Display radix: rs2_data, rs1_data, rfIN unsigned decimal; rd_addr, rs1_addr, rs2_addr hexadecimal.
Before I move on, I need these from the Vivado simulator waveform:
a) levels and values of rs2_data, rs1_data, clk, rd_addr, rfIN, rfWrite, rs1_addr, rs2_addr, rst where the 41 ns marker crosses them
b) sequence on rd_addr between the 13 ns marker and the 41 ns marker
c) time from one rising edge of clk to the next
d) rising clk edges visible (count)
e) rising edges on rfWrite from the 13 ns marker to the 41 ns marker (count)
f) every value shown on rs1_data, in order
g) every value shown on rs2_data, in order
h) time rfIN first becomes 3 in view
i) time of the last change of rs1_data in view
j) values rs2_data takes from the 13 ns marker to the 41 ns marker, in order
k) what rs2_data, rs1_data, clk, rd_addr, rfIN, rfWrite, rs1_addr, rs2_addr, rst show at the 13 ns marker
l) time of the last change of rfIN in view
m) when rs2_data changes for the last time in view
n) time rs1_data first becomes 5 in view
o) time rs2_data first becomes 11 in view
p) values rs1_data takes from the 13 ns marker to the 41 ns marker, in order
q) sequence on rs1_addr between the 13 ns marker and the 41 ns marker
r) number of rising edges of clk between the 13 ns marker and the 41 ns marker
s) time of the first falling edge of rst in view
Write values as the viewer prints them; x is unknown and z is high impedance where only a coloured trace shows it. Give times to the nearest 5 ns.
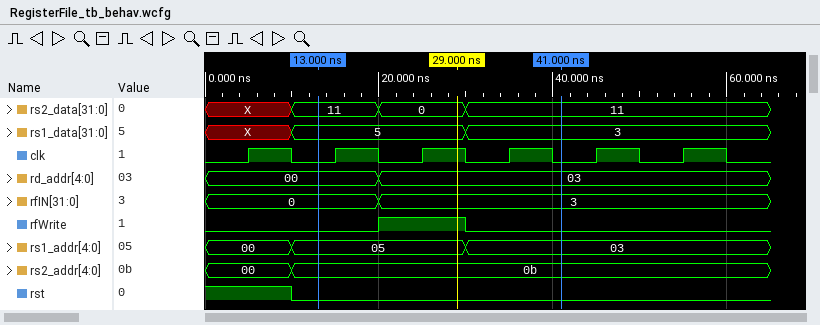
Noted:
rs2_data=11, rs1_data=3, clk=0, rd_addr=03, rfIN=3, rfWrite=0, rs1_addr=03, rs2_addr=0b, rst=0
00, 03
10 ns
6
1
X, 5, 3
X, 11, 0, 11
20 ns
30 ns
11, 0, 11
rs2_data=11, rs1_data=5, clk=0, rd_addr=00, rfIN=0, rfWrite=0, rs1_addr=05, rs2_addr=0b, rst=0
20 ns
30 ns
10 ns
10 ns
5, 3
05, 03
3
10 ns
